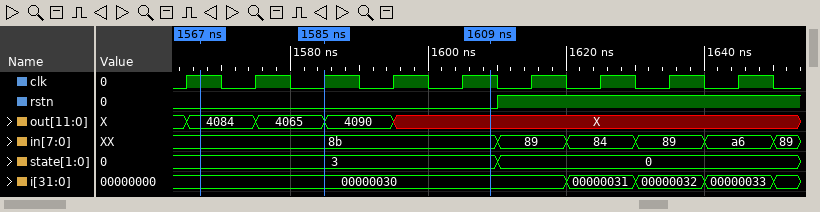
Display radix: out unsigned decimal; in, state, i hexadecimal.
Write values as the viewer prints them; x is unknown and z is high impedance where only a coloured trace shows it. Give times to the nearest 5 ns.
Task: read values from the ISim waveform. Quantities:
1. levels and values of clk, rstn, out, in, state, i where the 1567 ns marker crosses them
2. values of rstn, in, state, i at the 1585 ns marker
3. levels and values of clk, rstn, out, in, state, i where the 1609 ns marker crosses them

clk=1, rstn=0, out=4084, in=8b, state=3, i=00000030
rstn=0, in=8b, state=3, i=00000030
clk=1, rstn=0, out=X, in=8b, state=3, i=00000030
